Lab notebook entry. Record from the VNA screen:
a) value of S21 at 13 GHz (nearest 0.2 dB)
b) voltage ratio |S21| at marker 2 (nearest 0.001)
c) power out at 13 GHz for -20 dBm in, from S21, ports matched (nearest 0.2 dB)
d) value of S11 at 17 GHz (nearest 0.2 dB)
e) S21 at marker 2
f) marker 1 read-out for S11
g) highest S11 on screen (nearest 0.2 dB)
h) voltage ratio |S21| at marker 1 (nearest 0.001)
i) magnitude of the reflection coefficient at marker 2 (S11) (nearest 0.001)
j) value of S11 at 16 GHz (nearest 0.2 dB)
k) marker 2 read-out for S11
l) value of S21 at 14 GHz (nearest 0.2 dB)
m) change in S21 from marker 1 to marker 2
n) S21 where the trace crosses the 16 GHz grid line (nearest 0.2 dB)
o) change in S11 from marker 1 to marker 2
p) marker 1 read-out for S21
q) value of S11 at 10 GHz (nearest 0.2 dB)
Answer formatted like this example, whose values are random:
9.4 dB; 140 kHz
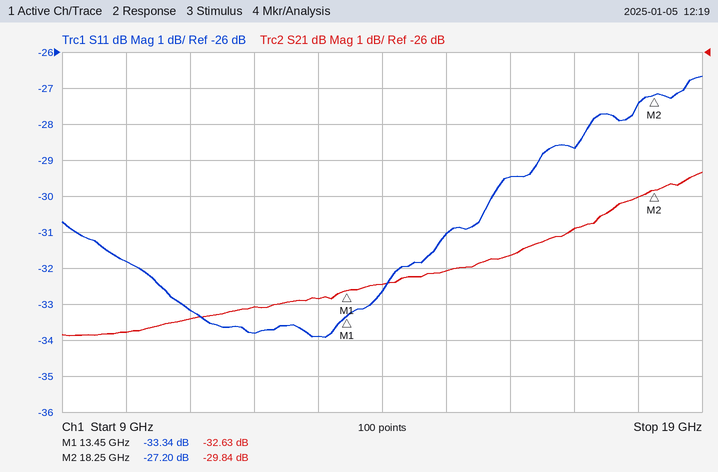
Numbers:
-32.8 dB; 0.032; -52.8 dBm; -28.6 dB; -29.84 dB; -33.34 dB; -26.6 dB; 0.023; 0.044; -29.4 dB; -27.20 dB; -32.4 dB; 2.79 dB; -31.6 dB; 6.14 dB; -32.63 dB; -31.8 dB
